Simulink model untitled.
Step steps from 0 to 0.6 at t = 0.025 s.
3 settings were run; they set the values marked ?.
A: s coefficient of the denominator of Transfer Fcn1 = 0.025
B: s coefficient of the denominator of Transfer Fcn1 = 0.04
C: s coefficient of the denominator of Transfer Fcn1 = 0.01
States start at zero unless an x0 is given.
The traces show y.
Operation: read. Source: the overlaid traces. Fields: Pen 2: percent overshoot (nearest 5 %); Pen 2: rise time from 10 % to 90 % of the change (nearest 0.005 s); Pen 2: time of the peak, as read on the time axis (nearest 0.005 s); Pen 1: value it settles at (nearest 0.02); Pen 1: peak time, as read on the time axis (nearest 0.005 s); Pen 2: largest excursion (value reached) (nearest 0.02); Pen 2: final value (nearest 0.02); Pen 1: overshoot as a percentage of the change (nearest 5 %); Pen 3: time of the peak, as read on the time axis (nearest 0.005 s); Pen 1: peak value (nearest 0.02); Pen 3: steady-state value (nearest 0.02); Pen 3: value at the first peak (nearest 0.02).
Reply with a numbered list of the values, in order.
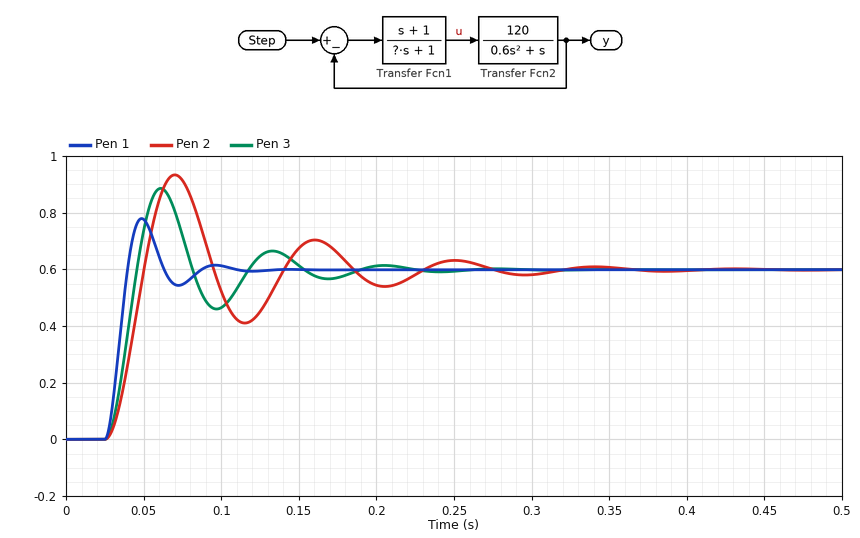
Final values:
1. 55 %
2. 0.015 s
3. 0.070 s
4. 0.60
5. 0.050 s
6. 0.94
7. 0.60
8. 30 %
9. 0.060 s
10. 0.78
11. 0.60
12. 0.88
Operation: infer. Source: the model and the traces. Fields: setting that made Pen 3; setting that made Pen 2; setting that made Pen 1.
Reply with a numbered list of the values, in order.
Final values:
1. A
2. B
3. C
